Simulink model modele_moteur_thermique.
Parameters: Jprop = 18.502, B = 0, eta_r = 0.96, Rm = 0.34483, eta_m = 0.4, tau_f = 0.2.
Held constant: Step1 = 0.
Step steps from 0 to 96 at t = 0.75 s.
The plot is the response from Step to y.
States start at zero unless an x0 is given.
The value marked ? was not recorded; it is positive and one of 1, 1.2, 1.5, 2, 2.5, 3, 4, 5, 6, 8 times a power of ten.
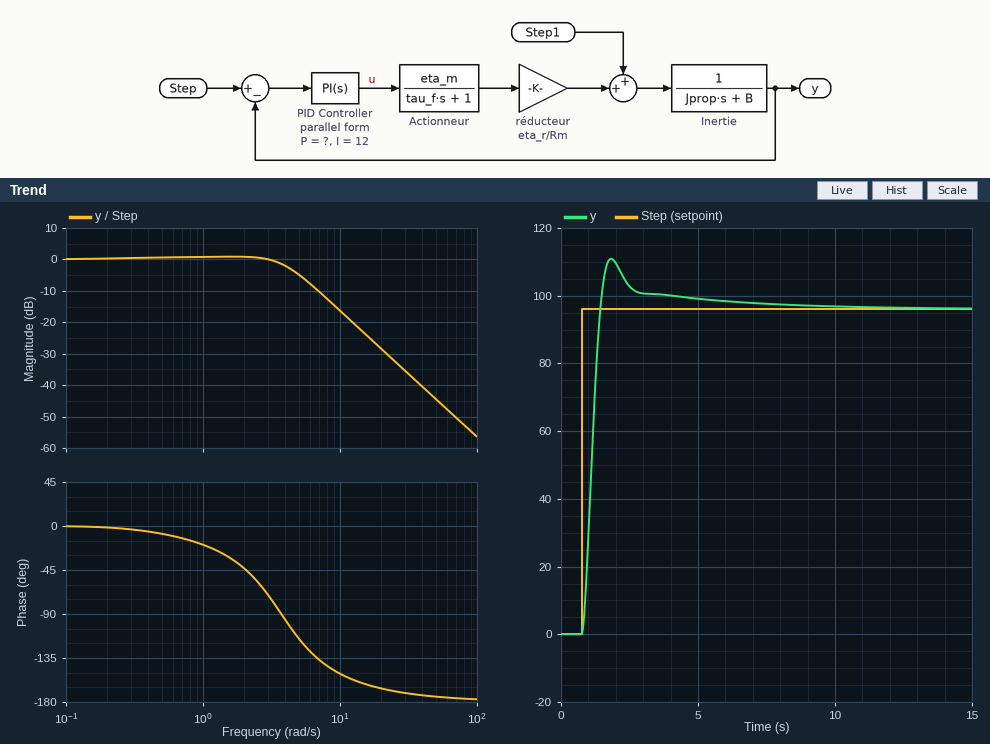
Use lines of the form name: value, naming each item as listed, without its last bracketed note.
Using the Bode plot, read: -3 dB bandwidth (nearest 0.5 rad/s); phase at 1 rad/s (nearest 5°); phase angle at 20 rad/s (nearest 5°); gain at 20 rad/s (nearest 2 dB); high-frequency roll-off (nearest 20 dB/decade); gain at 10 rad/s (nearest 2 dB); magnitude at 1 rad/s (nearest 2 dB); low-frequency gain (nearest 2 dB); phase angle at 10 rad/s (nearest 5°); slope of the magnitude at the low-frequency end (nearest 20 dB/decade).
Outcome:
-3 dB bandwidth: 4.5 rad/s
phase at 1 rad/s: -20°
phase angle at 20 rad/s: -165°
gain at 20 rad/s: -28 dB
high-frequency roll-off: -40 dB/decade
gain at 10 rad/s: -16 dB
magnitude at 1 rad/s: 0 dB
low-frequency gain: 0 dB
phase angle at 10 rad/s: -150°
slope of the magnitude at the low-frequency end: 0 dB/decade
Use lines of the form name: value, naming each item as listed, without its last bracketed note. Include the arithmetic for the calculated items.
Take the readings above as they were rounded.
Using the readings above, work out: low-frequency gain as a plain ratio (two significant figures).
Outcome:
low-frequency gain as a plain ratio: 10^(0 / 20) = 1.0
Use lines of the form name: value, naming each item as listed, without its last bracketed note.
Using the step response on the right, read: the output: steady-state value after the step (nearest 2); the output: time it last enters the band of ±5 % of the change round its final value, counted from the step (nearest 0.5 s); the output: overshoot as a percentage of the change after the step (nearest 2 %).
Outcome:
the output: steady-state value after the step: 96
the output: time it last enters the band of ±5 % of the change round its final value, counted from the step: 2.0 s
the output: overshoot as a percentage of the change after the step: 16 %
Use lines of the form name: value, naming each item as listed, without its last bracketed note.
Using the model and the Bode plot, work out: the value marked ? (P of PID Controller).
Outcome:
the value marked ?: 50
